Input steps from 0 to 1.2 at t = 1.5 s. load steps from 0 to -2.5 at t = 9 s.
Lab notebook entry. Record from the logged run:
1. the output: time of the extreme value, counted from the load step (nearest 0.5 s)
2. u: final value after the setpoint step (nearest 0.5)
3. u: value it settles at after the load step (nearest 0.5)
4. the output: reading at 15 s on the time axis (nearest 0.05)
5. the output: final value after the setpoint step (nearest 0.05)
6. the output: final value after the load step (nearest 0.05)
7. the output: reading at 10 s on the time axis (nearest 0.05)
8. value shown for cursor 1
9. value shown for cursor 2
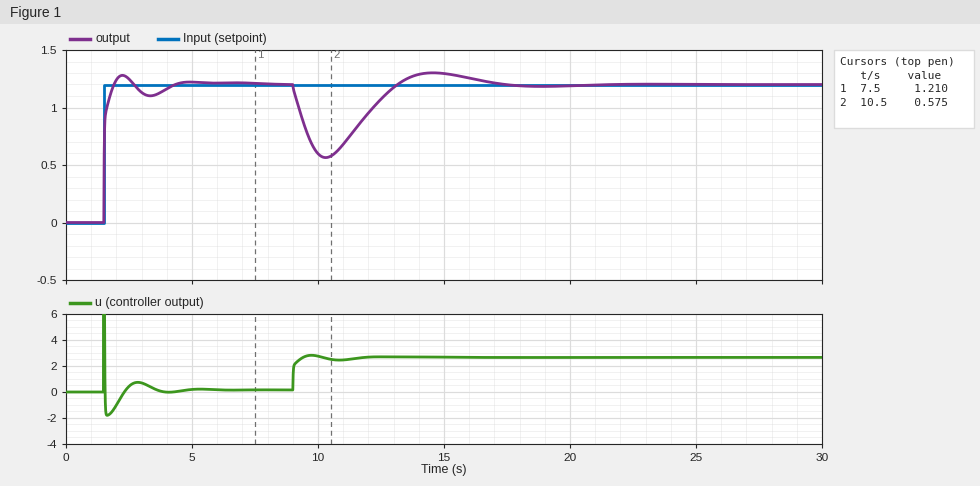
1.5 s
0.0
2.5
1.30
1.20
1.20
0.60
1.210
0.575
